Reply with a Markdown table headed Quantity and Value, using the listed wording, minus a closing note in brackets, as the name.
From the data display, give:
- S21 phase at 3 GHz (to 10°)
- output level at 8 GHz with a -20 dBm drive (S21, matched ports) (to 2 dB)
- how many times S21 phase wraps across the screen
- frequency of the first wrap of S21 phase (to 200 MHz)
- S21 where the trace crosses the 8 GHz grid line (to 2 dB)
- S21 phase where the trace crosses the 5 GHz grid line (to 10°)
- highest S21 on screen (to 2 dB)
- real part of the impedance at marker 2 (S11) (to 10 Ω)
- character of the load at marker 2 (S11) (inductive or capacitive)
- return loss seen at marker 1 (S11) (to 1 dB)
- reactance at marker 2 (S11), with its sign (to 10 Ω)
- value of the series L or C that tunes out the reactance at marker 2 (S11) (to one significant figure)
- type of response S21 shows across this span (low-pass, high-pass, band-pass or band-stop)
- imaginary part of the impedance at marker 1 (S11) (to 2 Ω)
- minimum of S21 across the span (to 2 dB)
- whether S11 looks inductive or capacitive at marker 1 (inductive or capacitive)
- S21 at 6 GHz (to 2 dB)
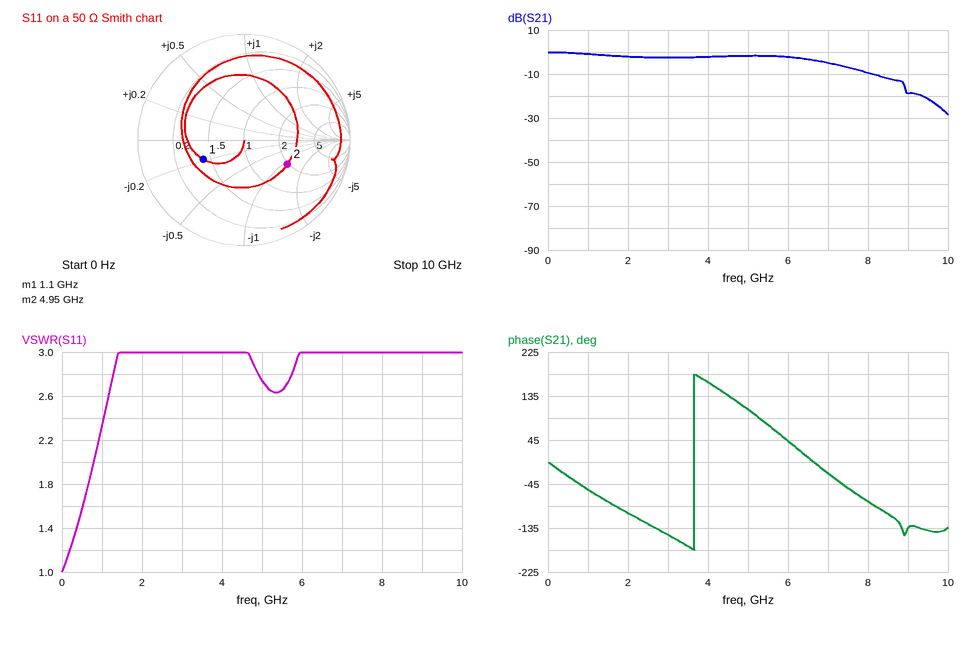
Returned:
| Quantity | Value |
|---|---|
| S21 phase at 3 GHz | -150° |
| output level at 8 GHz with a -20 dBm drive (S21, matched ports) | -30 dBm |
| how many times S21 phase wraps across the screen | 1 |
| frequency of the first wrap of S21 phase | 3.6 GHz |
| S21 where the trace crosses the 8 GHz grid line | -10 dB |
| S21 phase where the trace crosses the 5 GHz grid line | 110° |
| highest S21 on screen | 0 dB |
| real part of the impedance at marker 2 (S11) | 100 Ω |
| character of the load at marker 2 (S11) | capacitive |
| return loss seen at marker 1 (S11) | 7 dB |
| reactance at marker 2 (S11), with its sign | -60 Ω |
| value of the series L or C that tunes out the reactance at marker 2 (S11) | 2 nH |
| type of response S21 shows across this span | low-pass |
| imaginary part of the impedance at marker 1 (S11) | -10 Ω |
| minimum of S21 across the span | -28 dB |
| whether S11 looks inductive or capacitive at marker 1 | capacitive |
| S21 at 6 GHz | -2 dB |
